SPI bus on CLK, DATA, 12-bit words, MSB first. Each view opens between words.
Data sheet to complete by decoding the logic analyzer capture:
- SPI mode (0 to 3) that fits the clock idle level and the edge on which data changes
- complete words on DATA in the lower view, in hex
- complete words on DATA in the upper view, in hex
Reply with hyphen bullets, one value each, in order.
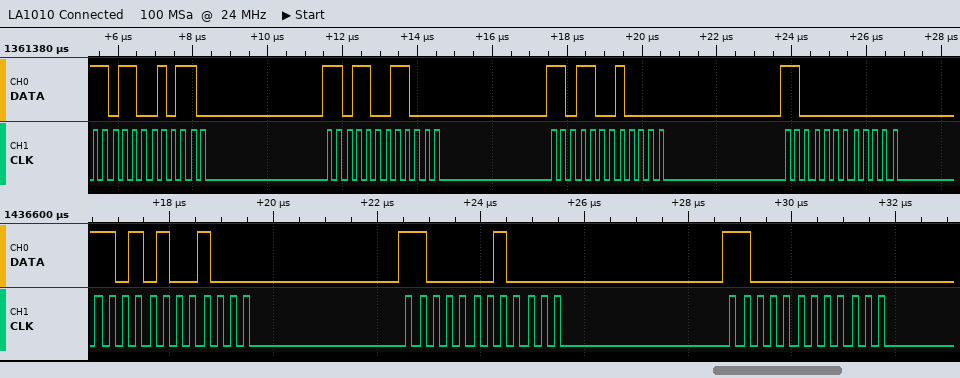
- 0
- D48, C10, C00
- D96, D98, D90, C00
